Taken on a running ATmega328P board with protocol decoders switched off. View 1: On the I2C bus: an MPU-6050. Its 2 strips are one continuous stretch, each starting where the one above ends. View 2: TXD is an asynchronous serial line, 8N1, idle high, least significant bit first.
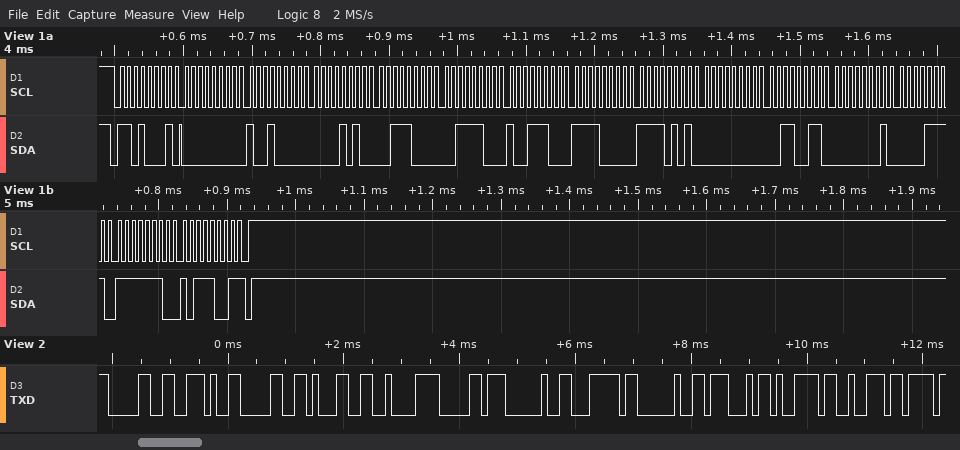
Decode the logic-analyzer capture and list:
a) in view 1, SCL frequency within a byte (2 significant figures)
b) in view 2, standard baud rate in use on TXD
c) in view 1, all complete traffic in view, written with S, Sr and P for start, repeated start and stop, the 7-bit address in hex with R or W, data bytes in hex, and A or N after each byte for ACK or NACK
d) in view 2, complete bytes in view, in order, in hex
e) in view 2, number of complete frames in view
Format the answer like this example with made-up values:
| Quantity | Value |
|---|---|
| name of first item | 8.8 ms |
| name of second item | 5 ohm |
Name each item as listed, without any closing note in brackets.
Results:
| Quantity | Value |
|---|---|
| in view 1, SCL frequency within a byte | 100 kHz |
| in view 2, standard baud rate in use on TXD | 9600 baud |
| in view 1, all complete traffic in view, written with S, Sr and P for start, repeated start and stop, the 7-bit address in hex with R or W, data bytes in hex, and A or N after each byte for ACK or NACK | S 68R A 00 A 90 A 0A A 38 A 3C A 9C A F0 A F5 A 00 A 33 A 01 A 0F A FE A B9 N P |
| in view 2, complete bytes in view, in order, in hex | 0x30 0x2E 0x30 0x31 0xC2 0xB0 0x20 0x7C 0x20 0x47 0x79 0x72 |
| in view 2, number of complete frames in view | 12 |
